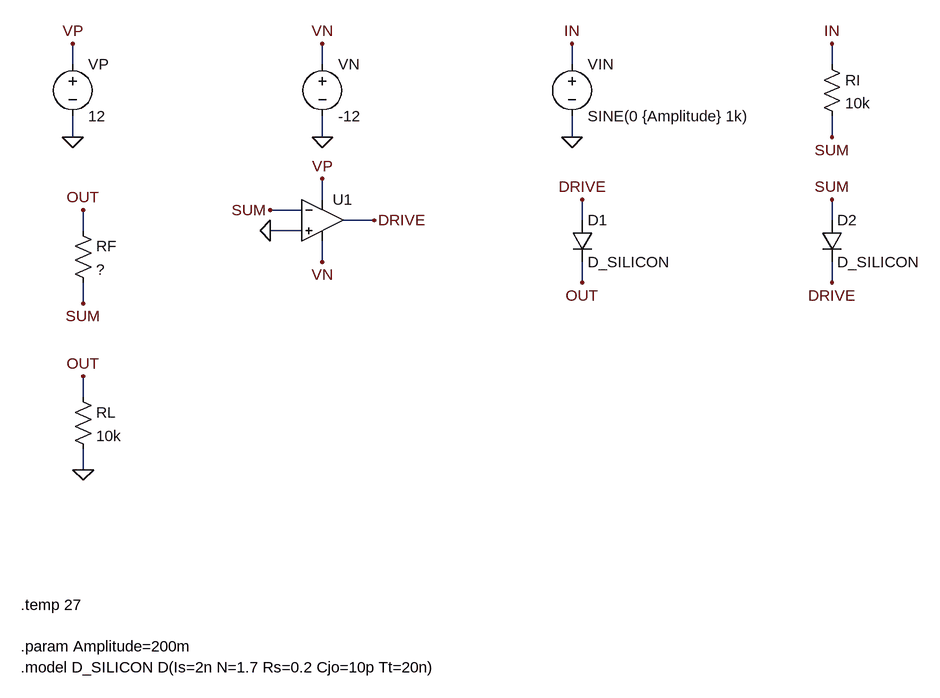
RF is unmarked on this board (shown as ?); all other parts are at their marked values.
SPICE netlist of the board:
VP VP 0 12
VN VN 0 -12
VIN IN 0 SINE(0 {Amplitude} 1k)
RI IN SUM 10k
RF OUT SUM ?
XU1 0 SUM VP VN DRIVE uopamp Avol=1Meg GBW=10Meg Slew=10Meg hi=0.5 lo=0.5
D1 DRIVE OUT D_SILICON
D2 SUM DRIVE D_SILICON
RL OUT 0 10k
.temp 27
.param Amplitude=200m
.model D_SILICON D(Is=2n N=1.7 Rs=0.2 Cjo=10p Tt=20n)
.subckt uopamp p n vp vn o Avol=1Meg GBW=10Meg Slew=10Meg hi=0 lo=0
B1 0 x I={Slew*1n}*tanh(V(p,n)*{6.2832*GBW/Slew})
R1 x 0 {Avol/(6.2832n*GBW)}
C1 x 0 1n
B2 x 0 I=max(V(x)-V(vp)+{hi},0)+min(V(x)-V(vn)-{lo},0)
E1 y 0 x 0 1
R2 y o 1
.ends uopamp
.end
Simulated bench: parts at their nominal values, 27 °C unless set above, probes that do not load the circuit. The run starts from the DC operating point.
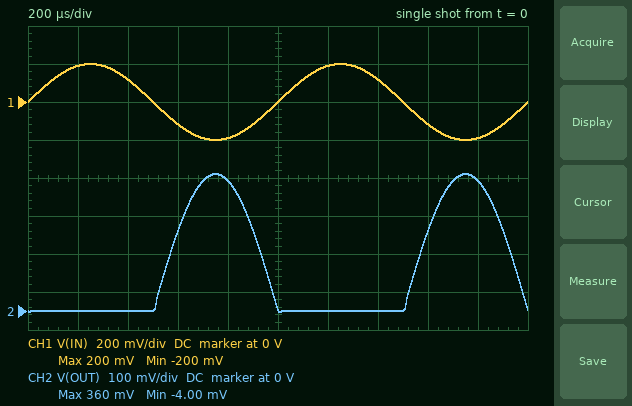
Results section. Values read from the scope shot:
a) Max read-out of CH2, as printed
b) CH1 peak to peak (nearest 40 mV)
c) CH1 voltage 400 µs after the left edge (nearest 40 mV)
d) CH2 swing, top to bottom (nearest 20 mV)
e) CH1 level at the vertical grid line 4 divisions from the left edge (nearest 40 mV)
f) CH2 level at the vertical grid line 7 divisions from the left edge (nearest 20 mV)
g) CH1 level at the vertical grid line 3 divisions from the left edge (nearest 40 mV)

360 mV
400 mV
120 mV
360 mV
-200 mV
0 V
-120 mV
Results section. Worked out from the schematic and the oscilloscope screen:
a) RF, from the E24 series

18 kΩ
